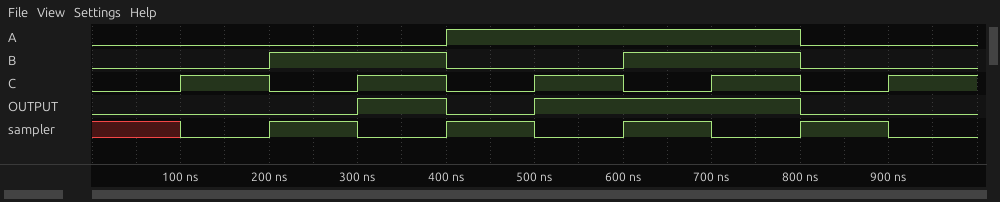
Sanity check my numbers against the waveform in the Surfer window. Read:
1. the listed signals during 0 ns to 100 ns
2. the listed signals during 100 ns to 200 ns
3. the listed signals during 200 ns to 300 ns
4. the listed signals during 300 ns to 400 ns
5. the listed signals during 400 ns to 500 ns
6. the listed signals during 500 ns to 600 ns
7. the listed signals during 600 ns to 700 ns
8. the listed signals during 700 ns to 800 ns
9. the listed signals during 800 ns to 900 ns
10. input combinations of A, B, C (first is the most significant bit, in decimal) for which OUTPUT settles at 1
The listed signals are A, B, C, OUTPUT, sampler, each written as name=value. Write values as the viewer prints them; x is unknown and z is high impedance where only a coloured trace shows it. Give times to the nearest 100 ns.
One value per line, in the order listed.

A=0, B=0, C=0, OUTPUT=0, sampler=x
A=0, B=0, C=1, OUTPUT=0, sampler=0
A=0, B=1, C=0, OUTPUT=0, sampler=1
A=0, B=1, C=1, OUTPUT=1, sampler=0
A=1, B=0, C=0, OUTPUT=0, sampler=1
A=1, B=0, C=1, OUTPUT=1, sampler=0
A=1, B=1, C=0, OUTPUT=1, sampler=1
A=1, B=1, C=1, OUTPUT=1, sampler=0
A=0, B=0, C=0, OUTPUT=0, sampler=1
3, 5, 6, 7
